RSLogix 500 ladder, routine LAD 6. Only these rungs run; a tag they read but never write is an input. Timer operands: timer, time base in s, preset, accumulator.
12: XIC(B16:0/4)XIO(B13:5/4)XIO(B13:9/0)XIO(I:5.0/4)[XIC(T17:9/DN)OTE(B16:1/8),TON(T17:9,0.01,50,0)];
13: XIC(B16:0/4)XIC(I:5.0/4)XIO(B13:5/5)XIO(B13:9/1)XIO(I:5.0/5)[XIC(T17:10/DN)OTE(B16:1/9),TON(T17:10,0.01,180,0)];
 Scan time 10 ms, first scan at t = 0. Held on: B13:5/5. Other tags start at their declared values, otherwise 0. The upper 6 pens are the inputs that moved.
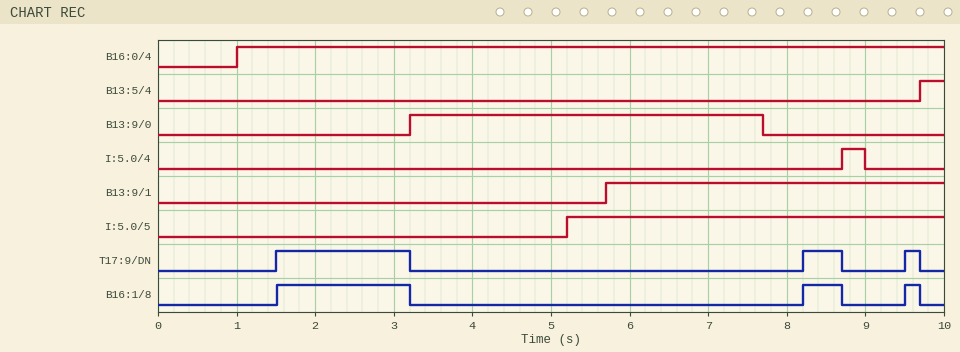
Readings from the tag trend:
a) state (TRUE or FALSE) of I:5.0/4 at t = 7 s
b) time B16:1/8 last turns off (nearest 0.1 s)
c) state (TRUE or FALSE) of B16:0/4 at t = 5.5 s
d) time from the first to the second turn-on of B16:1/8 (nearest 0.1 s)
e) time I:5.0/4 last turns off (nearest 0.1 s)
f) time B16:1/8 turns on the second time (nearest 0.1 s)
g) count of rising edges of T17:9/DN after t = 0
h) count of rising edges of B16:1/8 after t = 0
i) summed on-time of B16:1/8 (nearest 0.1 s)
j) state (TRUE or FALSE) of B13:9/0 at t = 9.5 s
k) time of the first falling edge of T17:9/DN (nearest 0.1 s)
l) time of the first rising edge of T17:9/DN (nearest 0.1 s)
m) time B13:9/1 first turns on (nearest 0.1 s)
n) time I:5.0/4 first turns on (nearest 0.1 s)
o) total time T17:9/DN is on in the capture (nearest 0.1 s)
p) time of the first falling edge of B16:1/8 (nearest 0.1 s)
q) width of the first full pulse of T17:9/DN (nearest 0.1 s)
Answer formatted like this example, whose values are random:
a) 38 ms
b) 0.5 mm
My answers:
a) FALSE
b) 9.7 s
c) TRUE
d) 6.7 s
e) 9.0 s
f) 8.2 s
g) 3
h) 3
i) 2.4 s
j) FALSE
k) 3.2 s
l) 1.5 s
m) 5.7 s
n) 8.7 s
o) 2.4 s
p) 3.2 s
q) 1.7 s
